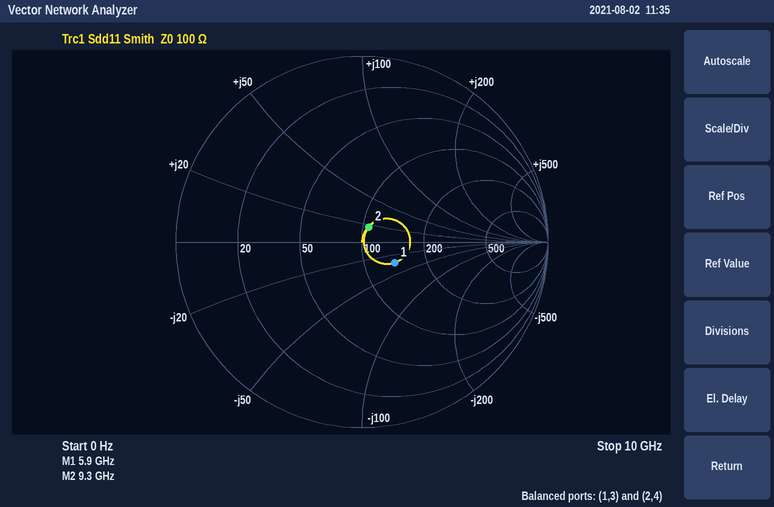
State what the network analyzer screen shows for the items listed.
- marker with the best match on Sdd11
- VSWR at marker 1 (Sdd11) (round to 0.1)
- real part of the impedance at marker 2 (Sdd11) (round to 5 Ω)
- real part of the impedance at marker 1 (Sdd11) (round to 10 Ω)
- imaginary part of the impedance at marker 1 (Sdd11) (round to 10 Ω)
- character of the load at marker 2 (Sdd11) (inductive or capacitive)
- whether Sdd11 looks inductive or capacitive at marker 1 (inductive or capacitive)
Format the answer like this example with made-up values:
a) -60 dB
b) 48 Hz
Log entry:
a) marker 2
b) 1.5
c) 105 Ω
d) 140 Ω
e) -30 Ω
f) inductive
g) capacitive
